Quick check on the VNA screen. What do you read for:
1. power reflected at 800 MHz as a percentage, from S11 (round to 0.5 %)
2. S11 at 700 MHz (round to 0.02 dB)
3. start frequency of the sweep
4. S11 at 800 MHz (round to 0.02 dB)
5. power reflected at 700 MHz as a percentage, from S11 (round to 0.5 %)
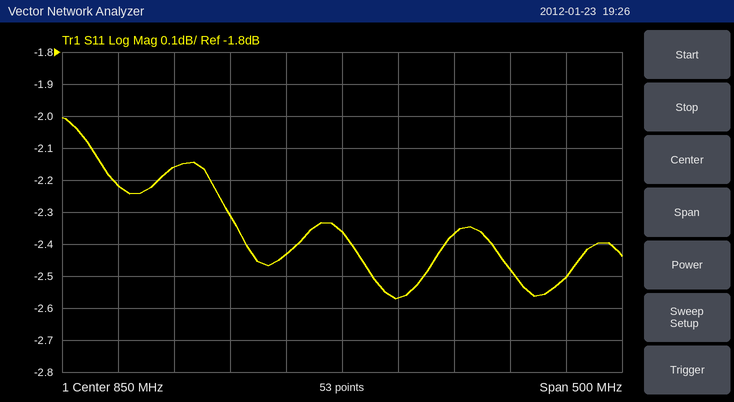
57.0 %
-2.16 dB
600 MHz
-2.44 dB
61.0 %
